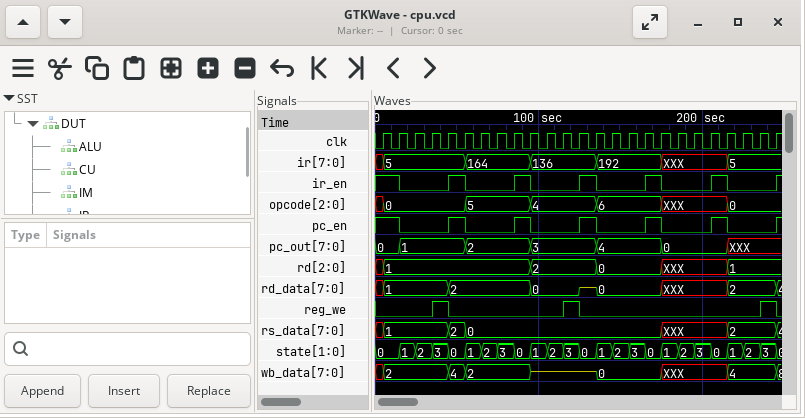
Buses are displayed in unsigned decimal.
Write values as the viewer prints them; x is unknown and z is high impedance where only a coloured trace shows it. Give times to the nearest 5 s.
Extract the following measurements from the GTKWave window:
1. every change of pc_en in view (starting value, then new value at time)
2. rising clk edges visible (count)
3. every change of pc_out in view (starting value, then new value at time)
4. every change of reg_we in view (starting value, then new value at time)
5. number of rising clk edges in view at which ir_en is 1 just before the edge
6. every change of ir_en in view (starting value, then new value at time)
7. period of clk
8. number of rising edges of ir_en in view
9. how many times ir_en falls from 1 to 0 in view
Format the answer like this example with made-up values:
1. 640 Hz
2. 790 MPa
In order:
1. 1, 0 at 15 s, 1 at 45 s, 0 at 55 s, 1 at 85 s, 0 at 95 s, 1 at 125 s, 0 at 135 s, 1 at 165 s, 0 at 175 s, 1 at 205 s, 0 at 215 s, 1 at 245 s
2. 25
3. 0, 1 at 15 s, 2 at 55 s, 3 at 95 s, 4 at 135 s, 0 at 175 s, XXX at 215 s
4. 0, 1 at 35 s, 0 at 45 s, 1 at 115 s, 0 at 125 s, 1 at 235 s, 0 at 245 s
5. 7
6. 1, 0 at 15 s, 1 at 45 s, 0 at 55 s, 1 at 85 s, 0 at 95 s, 1 at 125 s, 0 at 135 s, 1 at 165 s, 0 at 175 s, 1 at 205 s, 0 at 215 s, 1 at 245 s
7. 10 s
8. 6
9. 6
